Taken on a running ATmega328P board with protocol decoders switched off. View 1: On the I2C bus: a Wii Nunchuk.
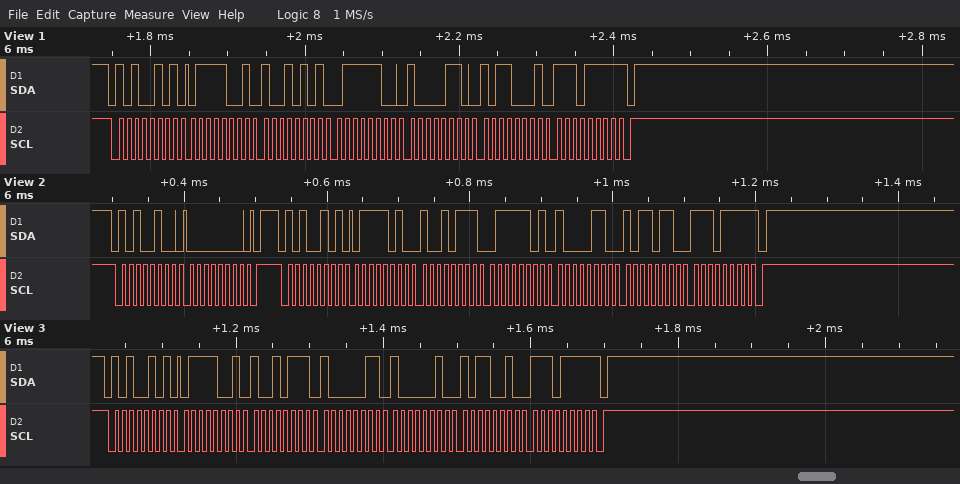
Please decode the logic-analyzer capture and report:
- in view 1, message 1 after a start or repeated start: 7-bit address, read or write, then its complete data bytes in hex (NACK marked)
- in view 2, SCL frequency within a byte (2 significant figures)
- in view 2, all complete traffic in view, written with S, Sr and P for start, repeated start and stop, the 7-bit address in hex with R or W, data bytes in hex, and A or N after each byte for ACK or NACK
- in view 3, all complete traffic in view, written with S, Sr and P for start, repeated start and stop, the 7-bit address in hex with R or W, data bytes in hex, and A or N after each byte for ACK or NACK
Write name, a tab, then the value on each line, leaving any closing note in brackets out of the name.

in view 1, message 1 after a start or repeated start: 7-bit address, read or write, then its complete data bytes in hex	0x52 read: 79 95 7C 86 B1 EF NACK
in view 2, SCL frequency within a byte	100 kHz
in view 2, all complete traffic in view, written with S, Sr and P for start, repeated start and stop, the 7-bit address in hex with R or W, data bytes in hex, and A or N after each byte for ACK or NACK	S 52W A 00 A P S 52R A 7A A 97 A 7D A 86 A B6 A EF N P
in view 3, all complete traffic in view, written with S, Sr and P for start, repeated start and stop, the 7-bit address in hex with R or W, data bytes in hex, and A or N after each byte for ACK or NACK	S 52R A 79 A 97 A 83 A 82 A B2 A EF N P
